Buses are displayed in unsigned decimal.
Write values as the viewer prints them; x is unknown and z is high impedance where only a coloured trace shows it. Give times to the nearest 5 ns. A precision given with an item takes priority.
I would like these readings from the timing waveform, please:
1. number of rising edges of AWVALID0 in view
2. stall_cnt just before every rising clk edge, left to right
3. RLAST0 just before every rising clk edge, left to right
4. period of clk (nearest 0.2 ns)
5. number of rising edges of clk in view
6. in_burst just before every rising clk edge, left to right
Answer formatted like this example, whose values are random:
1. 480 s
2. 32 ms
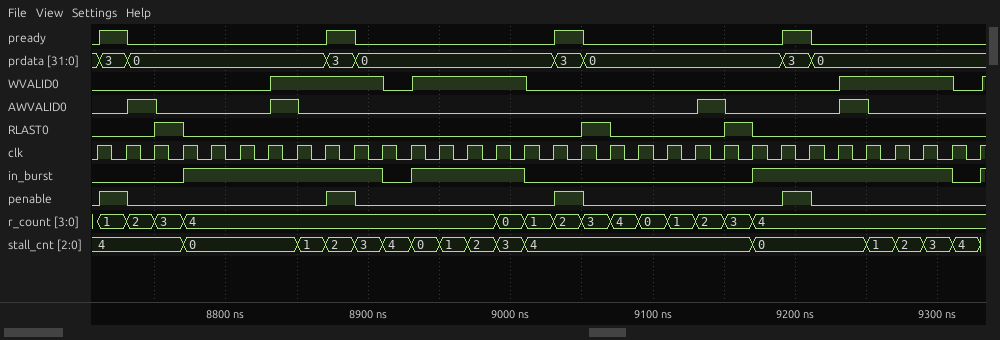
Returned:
1. 4
2. 4, 4, 4, 4, 0, 0, 0, 0, 1, 2, 3, 4, 0, 1, 2, 3, 4, 4, 4, 4, 4, 4, 4, 4, 0, 0, 0, 0, 1, 2, 3, 4
3. 0 0 0 1 0 0 0 0 0 0 0 0 0 0 0 0 0 0 1 0 0 0 0 1 0 0 0 0 0 0 0 0
4. 20 ns
5. 32
6. 0 0 0 0 1 1 1 1 1 1 1 0 1 1 1 1 0 0 0 0 0 0 0 0 1 1 1 1 1 1 1 0
